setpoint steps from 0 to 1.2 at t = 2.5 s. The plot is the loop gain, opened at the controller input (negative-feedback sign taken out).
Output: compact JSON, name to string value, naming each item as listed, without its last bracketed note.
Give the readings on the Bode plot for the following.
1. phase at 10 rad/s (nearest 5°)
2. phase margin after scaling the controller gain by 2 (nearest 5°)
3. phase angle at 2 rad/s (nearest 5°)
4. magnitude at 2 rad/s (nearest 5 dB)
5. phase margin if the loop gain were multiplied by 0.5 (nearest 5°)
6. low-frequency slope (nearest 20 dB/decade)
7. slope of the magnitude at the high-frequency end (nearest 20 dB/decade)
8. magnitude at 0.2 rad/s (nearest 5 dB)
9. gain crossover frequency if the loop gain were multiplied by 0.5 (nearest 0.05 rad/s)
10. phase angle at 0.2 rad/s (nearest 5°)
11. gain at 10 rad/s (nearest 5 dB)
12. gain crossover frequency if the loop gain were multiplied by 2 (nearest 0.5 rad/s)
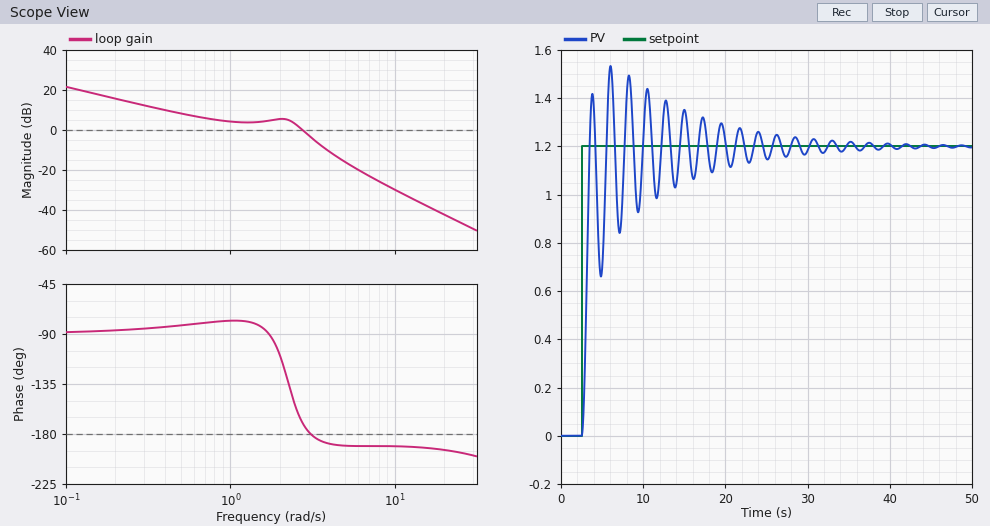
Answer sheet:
{"phase at 10 rad/s": "-190°", "phase margin after scaling the controller gain by 2": "-5°", "phase angle at 2 rad/s": "-110°", "magnitude at 2 rad/s": "5 dB", "phase margin if the loop gain were multiplied by 0.5": "100°", "low-frequency slope": "-20 dB/decade", "slope of the magnitude at the high-frequency end": "-40 dB/decade", "magnitude at 0.2 rad/s": "15 dB", "gain crossover frequency if the loop gain were multiplied by 0.5": "0.70 rad/s", "phase angle at 0.2 rad/s": "-85°", "gain at 10 rad/s": "-30 dB", "gain crossover frequency if the loop gain were multiplied by 2": "3.5 rad/s"}
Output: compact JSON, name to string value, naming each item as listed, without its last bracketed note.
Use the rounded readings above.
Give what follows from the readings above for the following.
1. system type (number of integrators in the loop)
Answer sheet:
{"system type": "1"}
